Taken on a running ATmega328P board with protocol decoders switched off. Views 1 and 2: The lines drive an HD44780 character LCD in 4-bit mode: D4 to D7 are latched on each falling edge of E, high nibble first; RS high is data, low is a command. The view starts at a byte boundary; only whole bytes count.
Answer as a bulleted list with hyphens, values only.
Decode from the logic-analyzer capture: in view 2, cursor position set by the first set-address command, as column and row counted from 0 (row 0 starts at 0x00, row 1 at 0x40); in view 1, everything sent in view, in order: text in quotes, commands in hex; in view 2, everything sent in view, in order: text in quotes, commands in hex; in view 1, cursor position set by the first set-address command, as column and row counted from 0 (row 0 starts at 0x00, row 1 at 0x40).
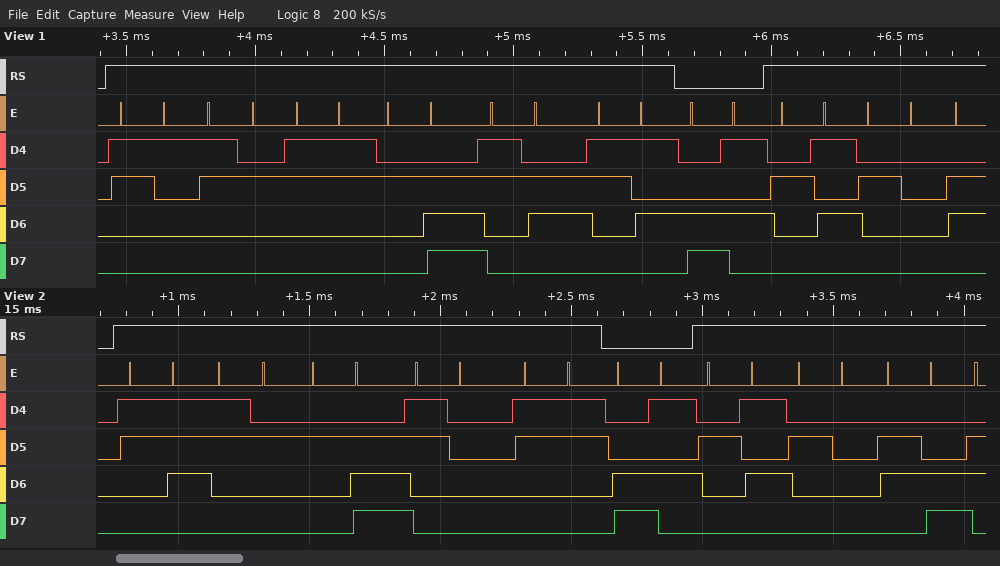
- column 5, row 1
- "123.65" 0xC5 "% "
- "72.03" 0xC5 "% l"
- column 5, row 1
